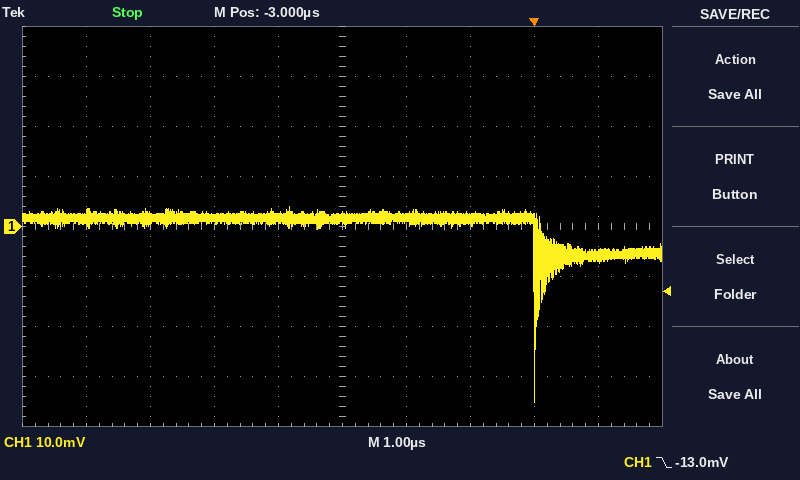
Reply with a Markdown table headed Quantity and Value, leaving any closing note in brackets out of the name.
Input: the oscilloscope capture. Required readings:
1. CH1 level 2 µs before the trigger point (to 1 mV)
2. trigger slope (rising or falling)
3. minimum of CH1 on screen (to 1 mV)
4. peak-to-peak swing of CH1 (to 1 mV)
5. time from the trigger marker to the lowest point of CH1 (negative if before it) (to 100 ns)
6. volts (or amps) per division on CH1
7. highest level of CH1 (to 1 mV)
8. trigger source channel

| Quantity | Value |
|---|---|
| CH1 level 2 µs before the trigger point | 2 mV |
| trigger slope | falling |
| minimum of CH1 on screen | -35 mV |
| peak-to-peak swing of CH1 | 39 mV |
| time from the trigger marker to the lowest point of CH1 (negative if before it) | 0.0 µs |
| volts (or amps) per division on CH1 | 10 mV |
| highest level of CH1 | 4 mV |
| trigger source channel | CH1 |
